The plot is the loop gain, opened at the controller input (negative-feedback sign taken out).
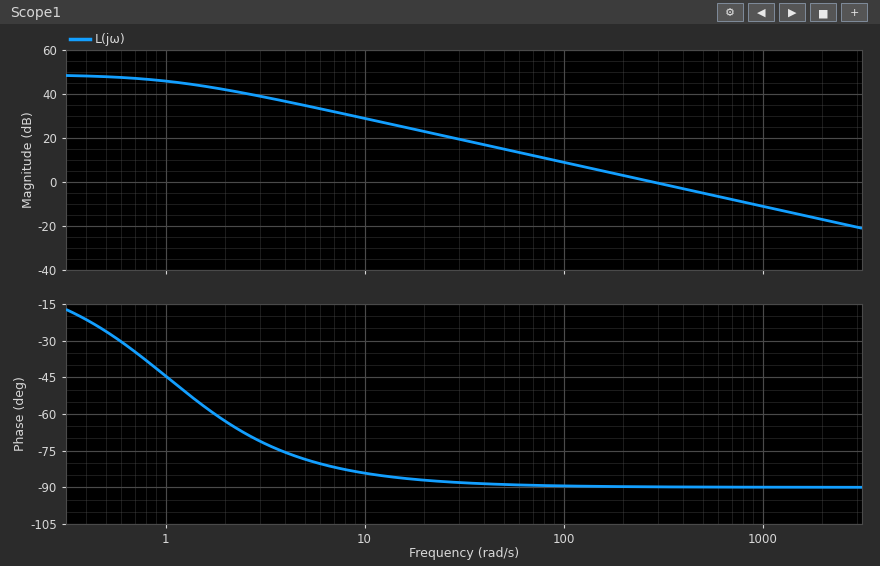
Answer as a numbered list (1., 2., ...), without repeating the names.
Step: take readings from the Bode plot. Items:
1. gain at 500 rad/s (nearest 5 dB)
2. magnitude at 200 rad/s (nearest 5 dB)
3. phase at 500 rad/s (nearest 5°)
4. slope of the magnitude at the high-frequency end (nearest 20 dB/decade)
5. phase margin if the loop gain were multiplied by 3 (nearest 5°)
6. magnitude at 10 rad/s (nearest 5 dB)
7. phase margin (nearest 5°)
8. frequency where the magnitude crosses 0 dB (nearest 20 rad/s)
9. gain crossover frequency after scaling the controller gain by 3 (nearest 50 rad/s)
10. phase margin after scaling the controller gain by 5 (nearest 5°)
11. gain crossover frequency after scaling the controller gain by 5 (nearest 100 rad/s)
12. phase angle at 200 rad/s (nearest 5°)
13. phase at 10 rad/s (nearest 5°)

1. -5 dB
2. 5 dB
3. -90°
4. -20 dB/decade
5. 90°
6. 30 dB
7. 90°
8. 280 rad/s
9. 850 rad/s
10. 90°
11. 1400 rad/s
12. -90°
13. -85°
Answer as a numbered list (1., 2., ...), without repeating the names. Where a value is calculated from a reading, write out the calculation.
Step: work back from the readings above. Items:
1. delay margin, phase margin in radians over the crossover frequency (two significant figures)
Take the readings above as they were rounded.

1. 90 × π / 180 / 280 = 0.0056 s
